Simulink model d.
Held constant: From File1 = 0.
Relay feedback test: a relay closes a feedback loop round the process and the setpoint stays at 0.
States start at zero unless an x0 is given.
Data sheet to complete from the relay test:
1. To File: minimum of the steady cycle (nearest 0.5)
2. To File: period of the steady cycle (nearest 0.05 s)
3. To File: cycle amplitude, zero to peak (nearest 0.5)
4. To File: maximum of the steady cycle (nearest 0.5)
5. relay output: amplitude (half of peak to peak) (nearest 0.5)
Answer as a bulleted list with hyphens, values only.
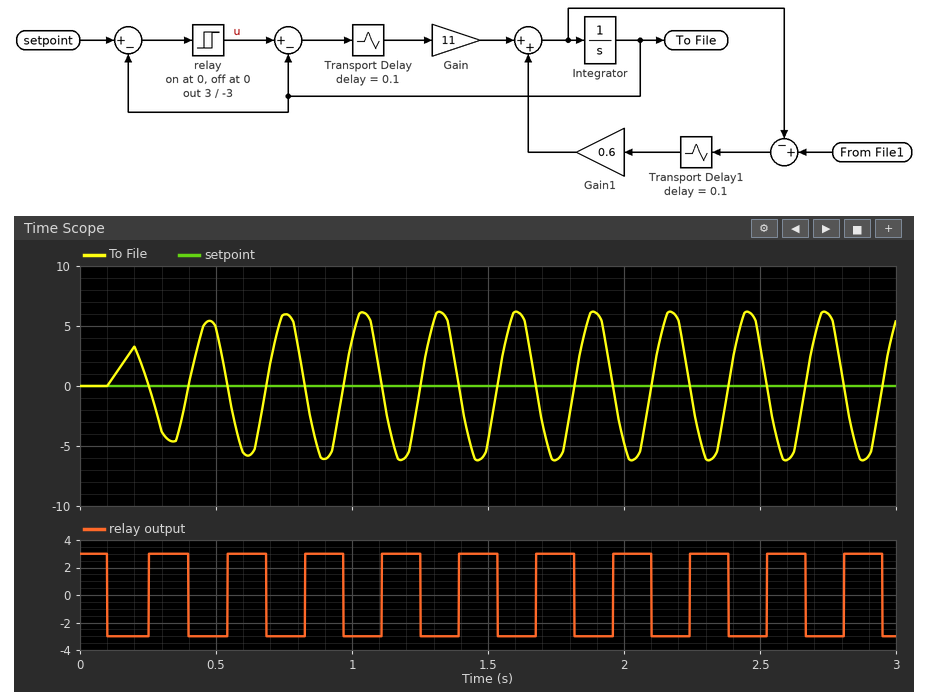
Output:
- -6.0
- 0.30 s
- 6.0
- 6.0
- 3.0
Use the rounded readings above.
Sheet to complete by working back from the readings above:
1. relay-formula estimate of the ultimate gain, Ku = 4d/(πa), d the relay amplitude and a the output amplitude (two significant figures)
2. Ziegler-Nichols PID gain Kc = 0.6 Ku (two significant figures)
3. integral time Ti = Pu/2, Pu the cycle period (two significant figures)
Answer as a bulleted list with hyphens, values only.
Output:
- 0.64
- 0.38
- 0.15 s
